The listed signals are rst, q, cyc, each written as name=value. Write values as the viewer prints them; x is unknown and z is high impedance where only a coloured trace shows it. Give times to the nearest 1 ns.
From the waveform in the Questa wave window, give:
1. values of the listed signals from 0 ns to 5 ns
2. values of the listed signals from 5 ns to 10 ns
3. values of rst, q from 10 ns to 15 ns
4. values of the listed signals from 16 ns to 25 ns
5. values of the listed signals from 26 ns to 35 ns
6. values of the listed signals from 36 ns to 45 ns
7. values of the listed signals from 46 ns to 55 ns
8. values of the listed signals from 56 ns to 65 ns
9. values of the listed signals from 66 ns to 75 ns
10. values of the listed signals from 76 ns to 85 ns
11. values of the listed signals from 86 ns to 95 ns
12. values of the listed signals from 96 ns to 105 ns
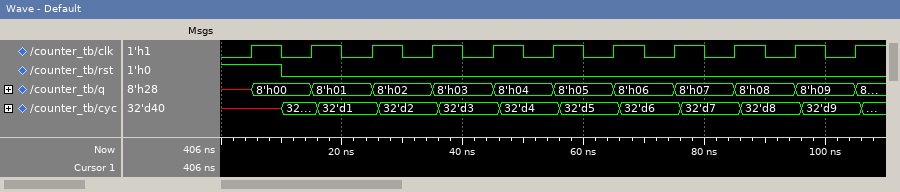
rst=1, q=x, cyc=x
rst=1, q=8'h00, cyc=x
rst=0, q=8'h00
rst=0, q=8'h01, cyc=32'd1
rst=0, q=8'h02, cyc=32'd2
rst=0, q=8'h03, cyc=32'd3
rst=0, q=8'h04, cyc=32'd4
rst=0, q=8'h05, cyc=32'd5
rst=0, q=8'h06, cyc=32'd6
rst=0, q=8'h07, cyc=32'd7
rst=0, q=8'h08, cyc=32'd8
rst=0, q=8'h09, cyc=32'd9
